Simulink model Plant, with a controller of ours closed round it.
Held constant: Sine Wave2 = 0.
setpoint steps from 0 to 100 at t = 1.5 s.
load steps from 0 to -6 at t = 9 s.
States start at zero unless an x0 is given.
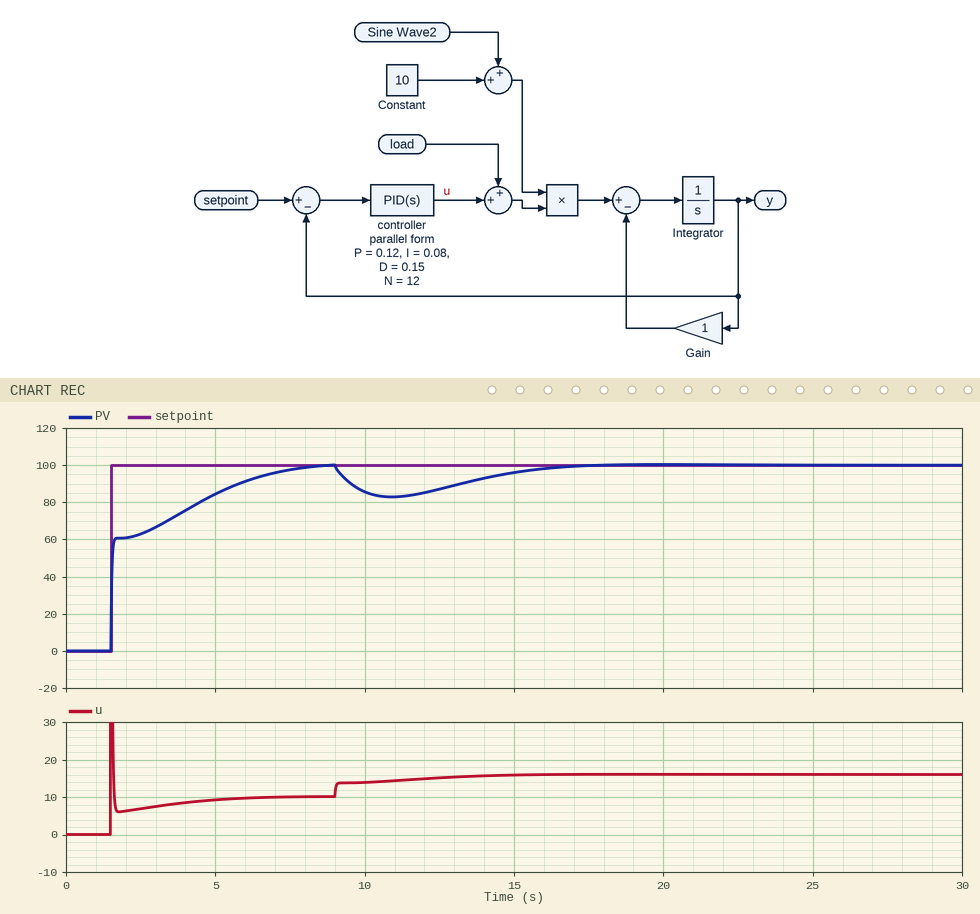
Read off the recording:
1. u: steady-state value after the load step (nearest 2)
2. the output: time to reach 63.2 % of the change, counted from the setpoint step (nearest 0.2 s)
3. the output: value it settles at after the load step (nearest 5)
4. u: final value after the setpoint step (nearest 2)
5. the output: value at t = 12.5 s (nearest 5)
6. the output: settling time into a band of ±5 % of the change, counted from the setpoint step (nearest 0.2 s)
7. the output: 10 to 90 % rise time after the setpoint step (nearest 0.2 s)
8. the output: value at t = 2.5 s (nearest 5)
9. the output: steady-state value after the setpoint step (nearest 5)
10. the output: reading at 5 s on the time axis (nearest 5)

16
1.0 s
100
10
85
5.2 s
4.2 s
65
100
85
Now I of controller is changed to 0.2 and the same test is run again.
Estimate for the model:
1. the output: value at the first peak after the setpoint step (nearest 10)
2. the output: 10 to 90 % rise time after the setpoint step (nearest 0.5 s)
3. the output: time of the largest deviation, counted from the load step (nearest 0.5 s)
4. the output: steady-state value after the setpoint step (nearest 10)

110
2.0 s
1.5 s
100
